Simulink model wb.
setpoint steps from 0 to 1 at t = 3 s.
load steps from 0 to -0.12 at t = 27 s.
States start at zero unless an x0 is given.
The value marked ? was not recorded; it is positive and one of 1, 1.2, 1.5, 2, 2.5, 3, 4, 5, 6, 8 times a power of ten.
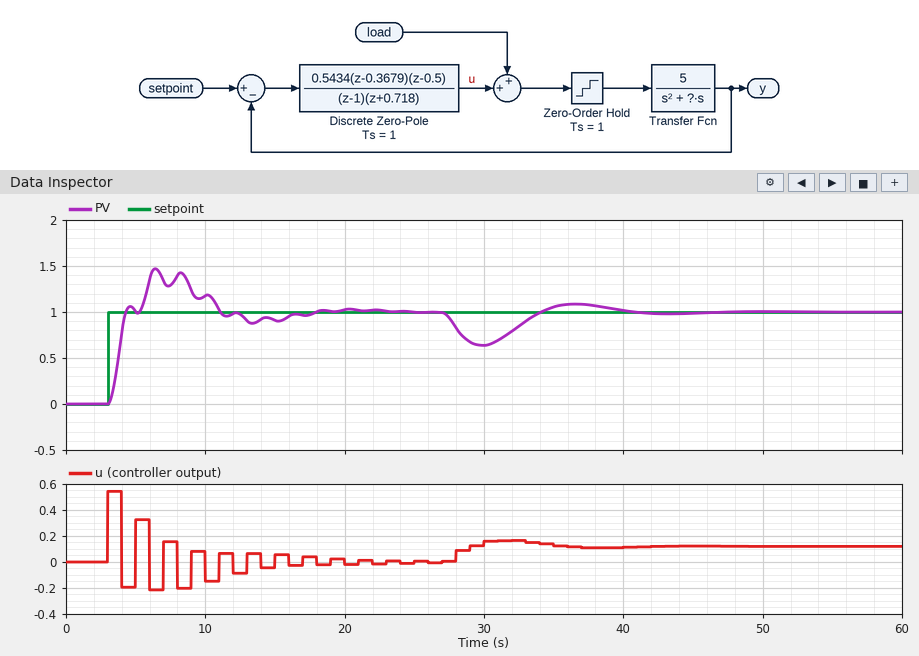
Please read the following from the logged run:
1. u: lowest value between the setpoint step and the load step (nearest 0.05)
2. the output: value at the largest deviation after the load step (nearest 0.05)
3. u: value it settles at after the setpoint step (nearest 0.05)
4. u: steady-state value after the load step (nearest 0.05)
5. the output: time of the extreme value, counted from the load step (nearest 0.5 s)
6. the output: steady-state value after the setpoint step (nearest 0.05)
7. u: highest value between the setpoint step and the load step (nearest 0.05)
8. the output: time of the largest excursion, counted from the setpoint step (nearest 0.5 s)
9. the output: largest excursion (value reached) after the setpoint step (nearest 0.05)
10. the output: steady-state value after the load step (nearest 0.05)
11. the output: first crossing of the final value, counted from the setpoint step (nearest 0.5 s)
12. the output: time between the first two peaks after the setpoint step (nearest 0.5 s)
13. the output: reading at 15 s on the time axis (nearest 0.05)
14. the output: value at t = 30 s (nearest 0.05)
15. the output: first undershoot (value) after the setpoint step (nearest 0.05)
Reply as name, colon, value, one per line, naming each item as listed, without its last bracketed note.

u: lowest value between the setpoint step and the load step: -0.20
the output: value at the largest deviation after the load step: 0.65
u: value it settles at after the setpoint step: 0.00
u: steady-state value after the load step: 0.10
the output: time of the extreme value, counted from the load step: 3.0 s
the output: steady-state value after the setpoint step: 1.00
u: highest value between the setpoint step and the load step: 0.55
the output: time of the largest excursion, counted from the setpoint step: 3.5 s
the output: largest excursion (value reached) after the setpoint step: 1.45
the output: steady-state value after the load step: 1.00
the output: first crossing of the final value, counted from the setpoint step: 1.5 s
the output: time between the first two peaks after the setpoint step: 2.0 s
the output: reading at 15 s on the time axis: 0.90
the output: value at t = 30 s: 0.65
the output: first undershoot (value) after the setpoint step: 1.30
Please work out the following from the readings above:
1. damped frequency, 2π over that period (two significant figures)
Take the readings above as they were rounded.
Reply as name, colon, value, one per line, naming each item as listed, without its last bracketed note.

damped frequency, 2π over that period: 3.1 rad/s
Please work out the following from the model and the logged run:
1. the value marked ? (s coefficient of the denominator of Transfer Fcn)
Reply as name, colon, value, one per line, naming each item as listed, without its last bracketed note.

the value marked ?: 2
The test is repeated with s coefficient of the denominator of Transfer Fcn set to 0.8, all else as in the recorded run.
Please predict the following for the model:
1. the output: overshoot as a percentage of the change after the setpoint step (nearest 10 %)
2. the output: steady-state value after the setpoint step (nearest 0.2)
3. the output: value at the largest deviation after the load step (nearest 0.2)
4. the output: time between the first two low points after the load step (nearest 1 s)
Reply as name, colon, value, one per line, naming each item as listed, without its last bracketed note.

the output: overshoot as a percentage of the change after the setpoint step: 70 %
the output: steady-state value after the setpoint step: 1.0
the output: value at the largest deviation after the load step: 0.4
the output: time between the first two low points after the load step: 7 s
